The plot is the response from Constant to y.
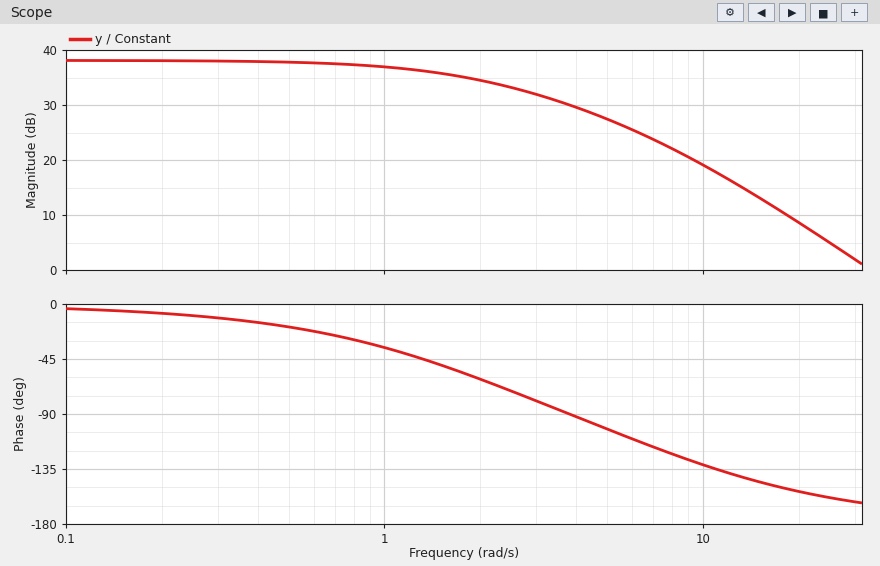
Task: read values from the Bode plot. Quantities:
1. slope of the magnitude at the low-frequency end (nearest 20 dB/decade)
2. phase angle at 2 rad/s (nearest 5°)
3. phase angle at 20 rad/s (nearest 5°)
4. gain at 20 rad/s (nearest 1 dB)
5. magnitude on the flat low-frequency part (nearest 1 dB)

0 dB/decade
-60°
-155°
9 dB
38 dB
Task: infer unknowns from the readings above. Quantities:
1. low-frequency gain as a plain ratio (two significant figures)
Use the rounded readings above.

79
